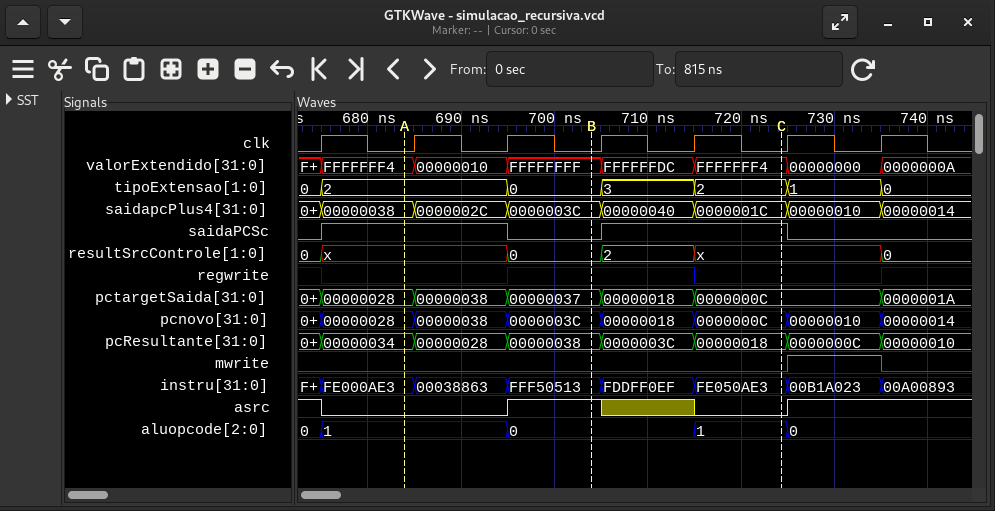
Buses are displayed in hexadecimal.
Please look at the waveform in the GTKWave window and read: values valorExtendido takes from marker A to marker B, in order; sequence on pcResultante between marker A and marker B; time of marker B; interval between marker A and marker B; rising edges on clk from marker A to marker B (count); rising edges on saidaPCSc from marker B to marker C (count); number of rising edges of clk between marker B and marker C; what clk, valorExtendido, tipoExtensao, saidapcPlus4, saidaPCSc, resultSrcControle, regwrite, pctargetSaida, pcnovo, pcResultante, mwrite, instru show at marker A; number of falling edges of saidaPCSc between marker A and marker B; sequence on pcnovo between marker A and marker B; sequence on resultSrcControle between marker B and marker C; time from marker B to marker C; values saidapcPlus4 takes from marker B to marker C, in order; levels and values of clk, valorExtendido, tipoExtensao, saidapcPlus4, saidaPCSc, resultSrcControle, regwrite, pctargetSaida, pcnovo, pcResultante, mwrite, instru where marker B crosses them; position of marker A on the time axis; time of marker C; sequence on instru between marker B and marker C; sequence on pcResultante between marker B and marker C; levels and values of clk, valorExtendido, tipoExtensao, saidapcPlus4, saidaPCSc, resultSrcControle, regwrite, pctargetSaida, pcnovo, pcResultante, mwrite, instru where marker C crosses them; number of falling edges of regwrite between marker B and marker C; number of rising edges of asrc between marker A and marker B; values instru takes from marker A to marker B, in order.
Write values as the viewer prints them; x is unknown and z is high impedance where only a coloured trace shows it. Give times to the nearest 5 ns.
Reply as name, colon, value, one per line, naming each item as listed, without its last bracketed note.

values valorExtendido takes from marker A to marker B, in order: FFFFFFF4, 00000010, FFFFFFFF
sequence on pcResultante between marker A and marker B: 00000034, 00000028, 00000038
time of marker B: 705 ns
interval between marker A and marker B: 20 ns
rising edges on clk from marker A to marker B: 2
rising edges on saidaPCSc from marker B to marker C: 1
number of rising edges of clk between marker B and marker C: 2
what clk, valorExtendido, tipoExtensao, saidapcPlus4, saidaPCSc, resultSrcControle, regwrite, pctargetSaida, pcnovo, pcResultante, mwrite, instru show at marker A: clk=0, valorExtendido=FFFFFFF4, tipoExtensao=2, saidapcPlus4=00000038, saidaPCSc=1, resultSrcControle=x, regwrite=0, pctargetSaida=00000028, pcnovo=00000028, pcResultante=00000034, mwrite=0, instru=FE000AE3
number of falling edges of saidaPCSc between marker A and marker B: 1
sequence on pcnovo between marker A and marker B: 00000028, 00000038, 0000003C
sequence on resultSrcControle between marker B and marker C: 0, 2, x
time from marker B to marker C: 20 ns
values saidapcPlus4 takes from marker B to marker C, in order: 0000003C, 00000040, 0000001C
levels and values of clk, valorExtendido, tipoExtensao, saidapcPlus4, saidaPCSc, resultSrcControle, regwrite, pctargetSaida, pcnovo, pcResultante, mwrite, instru where marker B crosses them: clk=0, valorExtendido=FFFFFFFF, tipoExtensao=0, saidapcPlus4=0000003C, saidaPCSc=0, resultSrcControle=0, regwrite=1, pctargetSaida=00000037, pcnovo=0000003C, pcResultante=00000038, mwrite=0, instru=FFF50513
position of marker A on the time axis: 685 ns
time of marker C: 725 ns
sequence on instru between marker B and marker C: FFF50513, FDDFF0EF, FE050AE3
sequence on pcResultante between marker B and marker C: 00000038, 0000003C, 00000018
levels and values of clk, valorExtendido, tipoExtensao, saidapcPlus4, saidaPCSc, resultSrcControle, regwrite, pctargetSaida, pcnovo, pcResultante, mwrite, instru where marker C crosses them: clk=0, valorExtendido=FFFFFFF4, tipoExtensao=2, saidapcPlus4=0000001C, saidaPCSc=1, resultSrcControle=x, regwrite=0, pctargetSaida=0000000C, pcnovo=0000000C, pcResultante=00000018, mwrite=0, instru=FE050AE3
number of falling edges of regwrite between marker B and marker C: 1
number of rising edges of asrc between marker A and marker B: 1
values instru takes from marker A to marker B, in order: FE000AE3, 00038863, FFF50513
